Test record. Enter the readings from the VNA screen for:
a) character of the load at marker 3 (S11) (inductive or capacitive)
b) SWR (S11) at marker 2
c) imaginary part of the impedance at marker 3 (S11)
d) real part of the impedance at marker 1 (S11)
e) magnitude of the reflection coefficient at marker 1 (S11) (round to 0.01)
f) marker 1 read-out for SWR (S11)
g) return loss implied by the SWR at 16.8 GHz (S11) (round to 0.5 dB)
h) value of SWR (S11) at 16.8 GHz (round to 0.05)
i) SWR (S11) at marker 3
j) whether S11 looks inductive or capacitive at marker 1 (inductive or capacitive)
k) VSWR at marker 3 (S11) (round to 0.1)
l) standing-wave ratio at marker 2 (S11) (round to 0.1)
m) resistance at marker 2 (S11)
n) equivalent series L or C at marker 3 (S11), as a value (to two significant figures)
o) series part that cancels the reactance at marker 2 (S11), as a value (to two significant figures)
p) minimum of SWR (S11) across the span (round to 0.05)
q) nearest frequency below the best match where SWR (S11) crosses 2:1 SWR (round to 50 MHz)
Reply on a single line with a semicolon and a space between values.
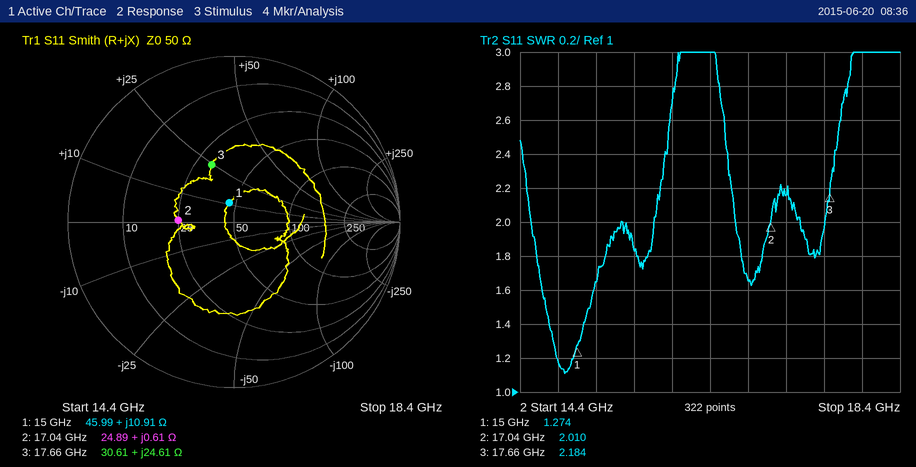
inductive; 2.010; +24.61 Ω; 45.99 Ω; 0.12; 1.274; 12.0 dB; 1.65; 2.184; inductive; 2.2; 2.0; 24.89 Ω; 220 pH; 15 pF; 1.10; 14.50 GHz
